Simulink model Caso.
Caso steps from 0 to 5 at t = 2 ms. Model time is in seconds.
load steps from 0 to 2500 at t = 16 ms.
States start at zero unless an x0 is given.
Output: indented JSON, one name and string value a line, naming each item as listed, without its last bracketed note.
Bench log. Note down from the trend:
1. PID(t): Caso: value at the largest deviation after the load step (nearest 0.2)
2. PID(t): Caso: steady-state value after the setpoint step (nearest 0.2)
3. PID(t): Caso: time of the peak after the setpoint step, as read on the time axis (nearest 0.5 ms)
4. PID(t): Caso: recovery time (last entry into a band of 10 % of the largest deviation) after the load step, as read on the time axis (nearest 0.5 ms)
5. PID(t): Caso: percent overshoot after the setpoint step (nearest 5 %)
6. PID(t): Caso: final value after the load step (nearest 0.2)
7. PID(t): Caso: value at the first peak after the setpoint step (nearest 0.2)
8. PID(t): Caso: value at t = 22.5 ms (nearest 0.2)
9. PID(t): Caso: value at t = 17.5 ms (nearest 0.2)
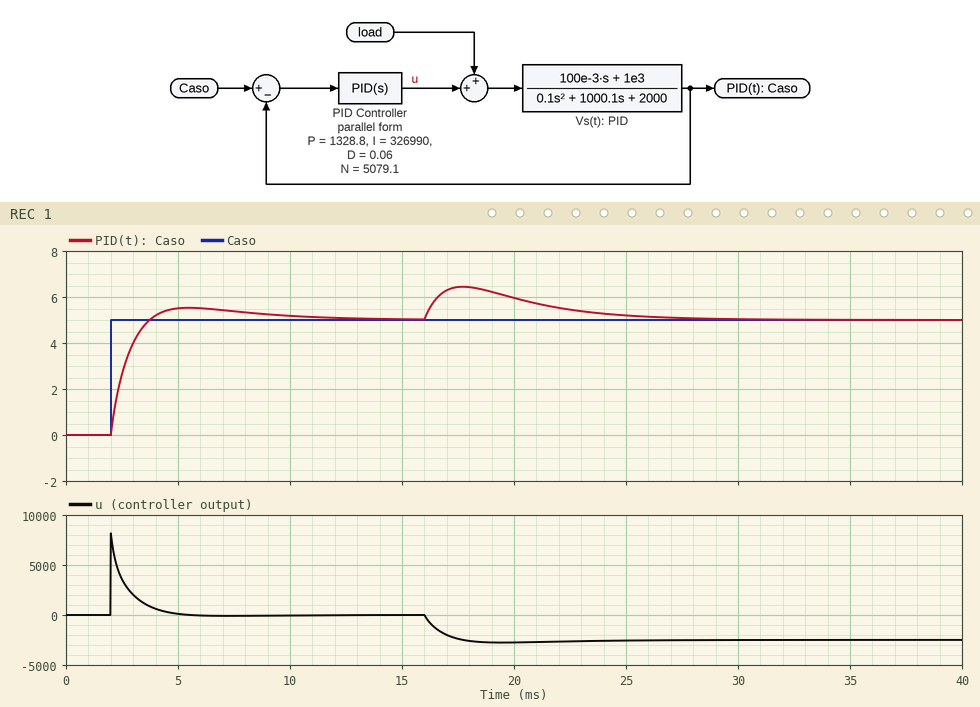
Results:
{
  "PID(t): Caso: value at the largest deviation after the load step": "6.4",
  "PID(t): Caso: steady-state value after the setpoint step": "5.0",
  "PID(t): Caso: time of the peak after the setpoint step, as read on the time axis": "5.5 ms",
  "PID(t): Caso: recovery time (last entry into a band of 10 % of the largest deviation) after the load step, as read on the time axis": "26.0 ms",
  "PID(t): Caso: percent overshoot after the setpoint step": "10 %",
  "PID(t): Caso: final value after the load step": "5.0",
  "PID(t): Caso: value at the first peak after the setpoint step": "5.6",
  "PID(t): Caso: value at t = 22.5 ms": "5.4",
  "PID(t): Caso: value at t = 17.5 ms": "6.4"
}
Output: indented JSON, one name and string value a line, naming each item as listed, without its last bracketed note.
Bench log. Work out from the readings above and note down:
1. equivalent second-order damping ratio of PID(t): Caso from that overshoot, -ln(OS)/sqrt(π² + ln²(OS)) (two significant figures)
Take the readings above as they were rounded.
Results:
{
  "equivalent second-order damping ratio of PID(t): Caso from that overshoot, -ln(OS)/sqrt(π² + ln²(OS))": "0.59"
}
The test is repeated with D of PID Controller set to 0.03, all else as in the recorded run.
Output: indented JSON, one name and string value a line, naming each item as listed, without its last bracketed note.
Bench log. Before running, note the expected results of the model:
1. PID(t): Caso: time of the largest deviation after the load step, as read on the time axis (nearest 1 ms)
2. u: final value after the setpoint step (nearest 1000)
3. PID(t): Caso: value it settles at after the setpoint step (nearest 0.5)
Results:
{
  "PID(t): Caso: time of the largest deviation after the load step, as read on the time axis": "18 ms",
  "u: final value after the setpoint step": "0",
  "PID(t): Caso: value it settles at after the setpoint step": "5.0"
}
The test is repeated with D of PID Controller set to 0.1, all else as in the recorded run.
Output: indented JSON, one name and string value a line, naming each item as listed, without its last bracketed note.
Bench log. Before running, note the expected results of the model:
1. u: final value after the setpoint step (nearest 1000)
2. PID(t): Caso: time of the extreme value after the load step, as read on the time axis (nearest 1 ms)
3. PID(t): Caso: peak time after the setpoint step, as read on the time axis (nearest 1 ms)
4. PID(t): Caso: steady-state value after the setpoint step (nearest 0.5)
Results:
{
  "u: final value after the setpoint step": "0",
  "PID(t): Caso: time of the extreme value after the load step, as read on the time axis": "18 ms",
  "PID(t): Caso: peak time after the setpoint step, as read on the time axis": "6 ms",
  "PID(t): Caso: steady-state value after the setpoint step": "5.0"
}
